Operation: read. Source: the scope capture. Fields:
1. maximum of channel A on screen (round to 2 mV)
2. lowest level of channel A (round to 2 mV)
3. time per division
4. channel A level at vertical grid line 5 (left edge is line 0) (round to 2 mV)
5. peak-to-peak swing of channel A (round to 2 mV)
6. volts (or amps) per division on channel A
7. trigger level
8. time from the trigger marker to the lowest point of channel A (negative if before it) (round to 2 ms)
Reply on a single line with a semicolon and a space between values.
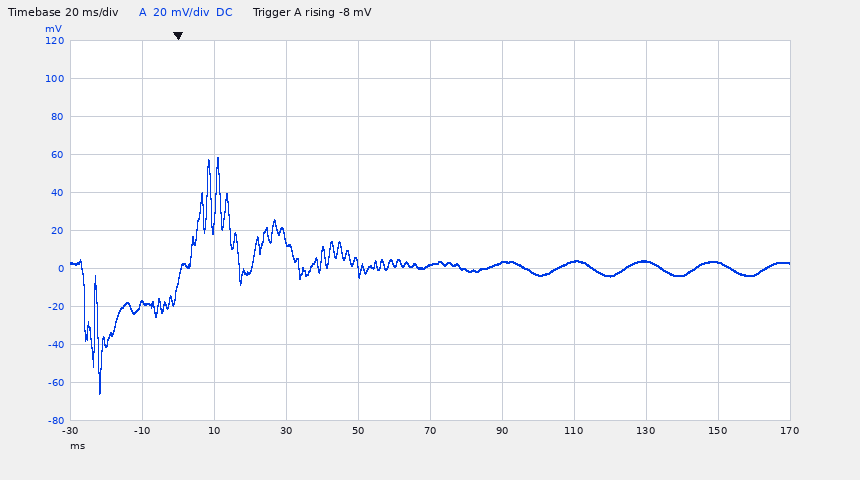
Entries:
58 mV; -66 mV; 20 ms; 2 mV; 124 mV; 20 mV; -8 mV; -22 ms
